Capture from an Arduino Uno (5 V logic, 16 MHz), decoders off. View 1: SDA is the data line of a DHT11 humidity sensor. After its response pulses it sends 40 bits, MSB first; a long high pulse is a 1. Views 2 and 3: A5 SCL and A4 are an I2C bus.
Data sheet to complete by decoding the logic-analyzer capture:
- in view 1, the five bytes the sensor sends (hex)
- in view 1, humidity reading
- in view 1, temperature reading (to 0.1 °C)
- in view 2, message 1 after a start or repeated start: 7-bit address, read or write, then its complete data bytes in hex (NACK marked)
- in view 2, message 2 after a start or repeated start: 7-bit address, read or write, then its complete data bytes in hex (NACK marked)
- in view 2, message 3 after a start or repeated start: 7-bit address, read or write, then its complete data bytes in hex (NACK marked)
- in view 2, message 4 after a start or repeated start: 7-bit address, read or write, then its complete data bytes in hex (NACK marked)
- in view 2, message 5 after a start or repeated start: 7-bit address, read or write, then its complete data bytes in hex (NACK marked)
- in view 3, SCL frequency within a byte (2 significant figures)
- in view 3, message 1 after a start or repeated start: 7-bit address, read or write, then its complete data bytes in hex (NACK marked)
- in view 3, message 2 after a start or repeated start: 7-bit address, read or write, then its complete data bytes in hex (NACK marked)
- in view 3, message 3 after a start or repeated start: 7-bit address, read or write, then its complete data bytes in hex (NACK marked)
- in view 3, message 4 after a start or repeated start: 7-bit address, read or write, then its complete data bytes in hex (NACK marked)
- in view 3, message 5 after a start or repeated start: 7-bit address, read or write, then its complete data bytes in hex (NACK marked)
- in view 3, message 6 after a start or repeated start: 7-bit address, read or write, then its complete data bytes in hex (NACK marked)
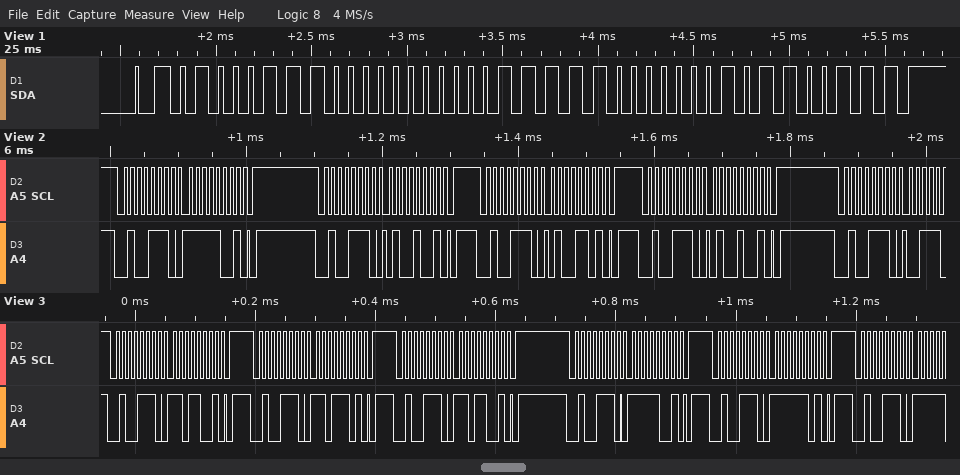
47 00 1F 01 67
71 %
31.1 °C
0x27 write: F9
0x27 write: 49
0x27 write: 4D
0x27 write: 49
0x27 write
100 kHz
0x27 write: D9
0x27 write: DD
0x27 write: D9
0x27 write: F9
0x27 write: FD
0x27 write
